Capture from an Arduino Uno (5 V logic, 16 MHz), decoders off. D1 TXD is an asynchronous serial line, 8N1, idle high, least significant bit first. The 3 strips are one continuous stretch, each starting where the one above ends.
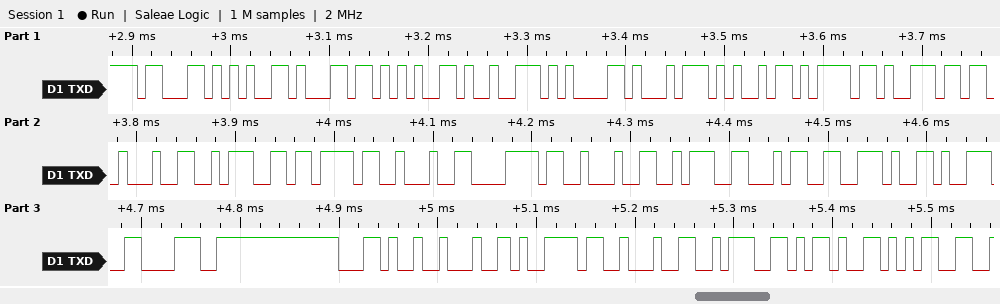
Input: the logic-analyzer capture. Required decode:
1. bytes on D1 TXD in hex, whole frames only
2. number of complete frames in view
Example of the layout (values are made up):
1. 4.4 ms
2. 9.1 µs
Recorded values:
1. 0x63 0x65 0x6C 0x65 0x72 0x61 0x74 0x69 0x6F 0x6E 0x22 0x3A 0x7B 0x22 0x78 0x22 0x3A 0x34 0x2E 0x39 0x38 0x2C 0x22 0x79 0x22 0x3A 0x2D 0x35
2. 28
